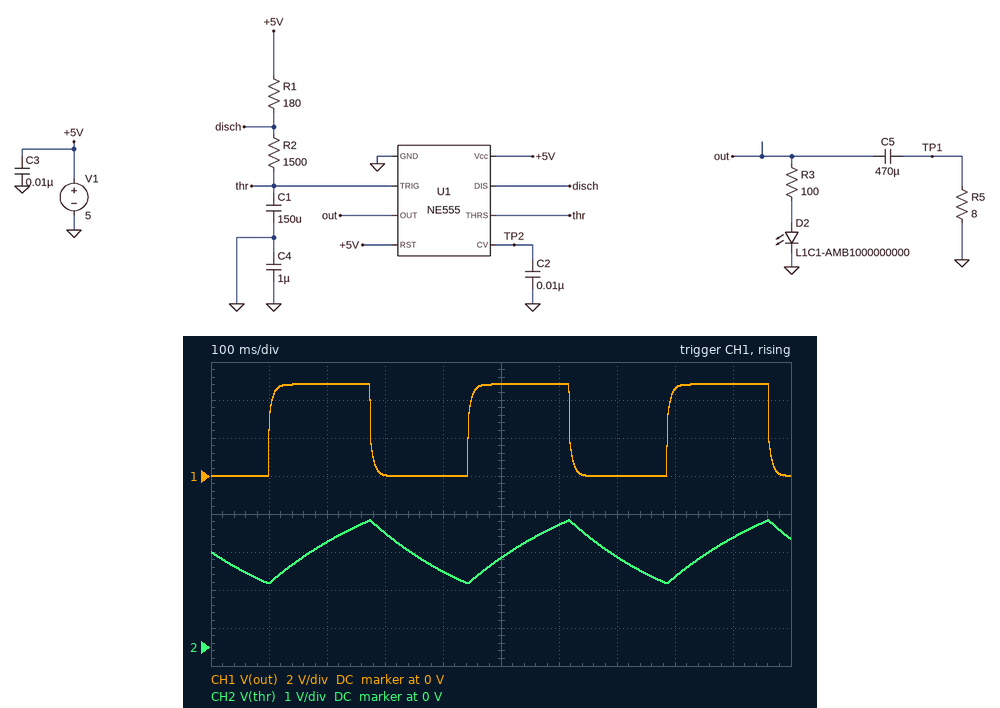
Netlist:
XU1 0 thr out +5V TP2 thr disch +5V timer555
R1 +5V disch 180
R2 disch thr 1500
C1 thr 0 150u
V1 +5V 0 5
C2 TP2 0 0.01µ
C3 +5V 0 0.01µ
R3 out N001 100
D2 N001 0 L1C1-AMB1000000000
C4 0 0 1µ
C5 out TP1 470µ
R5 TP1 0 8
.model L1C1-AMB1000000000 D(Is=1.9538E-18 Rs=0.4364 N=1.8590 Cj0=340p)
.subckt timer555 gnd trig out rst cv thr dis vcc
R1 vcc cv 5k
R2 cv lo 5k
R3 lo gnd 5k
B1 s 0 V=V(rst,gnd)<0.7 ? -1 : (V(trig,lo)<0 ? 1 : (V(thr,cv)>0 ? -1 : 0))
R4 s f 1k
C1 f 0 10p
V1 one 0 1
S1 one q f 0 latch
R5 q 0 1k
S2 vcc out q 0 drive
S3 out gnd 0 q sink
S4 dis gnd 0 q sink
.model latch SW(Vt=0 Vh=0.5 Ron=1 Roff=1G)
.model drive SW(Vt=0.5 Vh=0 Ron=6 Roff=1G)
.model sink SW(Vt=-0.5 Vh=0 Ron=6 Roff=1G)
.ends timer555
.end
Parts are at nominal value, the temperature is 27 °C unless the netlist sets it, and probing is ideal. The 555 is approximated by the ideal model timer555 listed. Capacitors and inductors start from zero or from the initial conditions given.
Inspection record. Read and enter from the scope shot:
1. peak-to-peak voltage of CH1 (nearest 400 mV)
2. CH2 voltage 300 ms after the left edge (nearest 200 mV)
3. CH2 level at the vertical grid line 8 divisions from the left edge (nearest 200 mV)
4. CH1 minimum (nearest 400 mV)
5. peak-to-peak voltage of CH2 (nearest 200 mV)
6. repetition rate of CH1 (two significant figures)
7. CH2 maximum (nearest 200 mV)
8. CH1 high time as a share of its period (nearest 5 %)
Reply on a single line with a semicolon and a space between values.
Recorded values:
4.8 V; 3.0 V; 1.8 V; 0 V; 1.6 V; 2.9 Hz; 3.4 V; 50 %
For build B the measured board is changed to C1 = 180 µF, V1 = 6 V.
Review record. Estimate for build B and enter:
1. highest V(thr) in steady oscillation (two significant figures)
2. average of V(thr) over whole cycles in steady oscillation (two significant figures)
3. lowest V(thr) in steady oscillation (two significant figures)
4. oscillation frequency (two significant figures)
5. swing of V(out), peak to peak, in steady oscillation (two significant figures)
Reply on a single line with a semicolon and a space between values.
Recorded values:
4.0 V; 3.0 V; 2.0 V; 2.4 Hz; 5.8 V
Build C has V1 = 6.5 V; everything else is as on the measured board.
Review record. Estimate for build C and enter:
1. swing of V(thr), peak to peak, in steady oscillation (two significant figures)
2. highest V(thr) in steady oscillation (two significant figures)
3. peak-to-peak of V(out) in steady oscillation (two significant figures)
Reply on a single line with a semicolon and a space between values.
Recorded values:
2.2 V; 4.3 V; 6.2 V
